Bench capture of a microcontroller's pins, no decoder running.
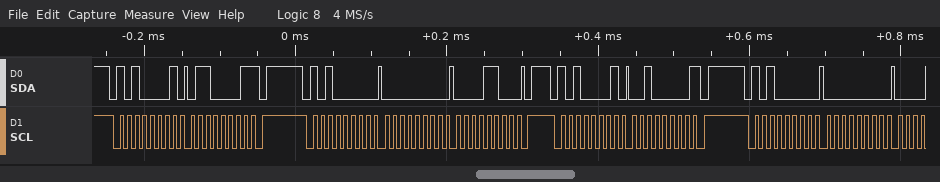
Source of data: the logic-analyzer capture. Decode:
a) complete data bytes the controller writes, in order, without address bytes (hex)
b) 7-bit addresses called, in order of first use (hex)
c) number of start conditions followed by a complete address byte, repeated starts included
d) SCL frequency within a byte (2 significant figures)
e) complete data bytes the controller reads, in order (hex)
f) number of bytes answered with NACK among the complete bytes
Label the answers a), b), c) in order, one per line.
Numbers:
a) 00 0C 00
b) 0x50
c) 4
d) 100 kHz
e) 61 20
f) 2
